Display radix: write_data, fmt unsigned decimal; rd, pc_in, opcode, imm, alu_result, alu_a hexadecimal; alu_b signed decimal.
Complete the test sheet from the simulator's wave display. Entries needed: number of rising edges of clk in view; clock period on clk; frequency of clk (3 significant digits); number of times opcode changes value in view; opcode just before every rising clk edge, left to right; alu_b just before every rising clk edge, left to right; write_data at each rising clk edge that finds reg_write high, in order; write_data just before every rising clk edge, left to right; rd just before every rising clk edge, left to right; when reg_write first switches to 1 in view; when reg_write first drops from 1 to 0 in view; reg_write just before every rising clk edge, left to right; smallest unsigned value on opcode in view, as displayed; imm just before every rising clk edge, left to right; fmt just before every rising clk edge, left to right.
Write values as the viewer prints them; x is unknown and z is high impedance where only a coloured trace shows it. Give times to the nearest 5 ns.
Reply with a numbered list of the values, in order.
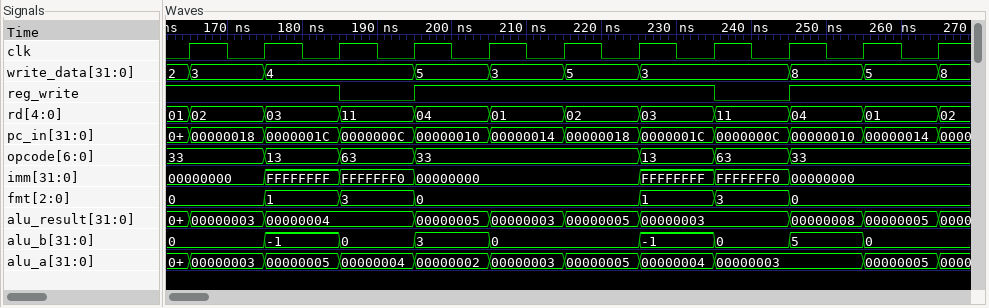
1. 11
2. 10 ns
3. 100 MHz
4. 6
5. 33, 33, 13, 63, 33, 33, 33, 13, 63, 33, 33
6. 0, 0, -1, 0, 3, 0, 0, -1, 0, 5, 0
7. 2, 3, 4, 5, 3, 5, 3, 8, 5
8. 2, 3, 4, 4, 5, 3, 5, 3, 3, 8, 5
9. 01, 02, 03, 11, 04, 01, 02, 03, 11, 04, 01
10. 195 ns
11. 185 ns
12. 1 1 1 0 1 1 1 1 0 1 1
13. 13
14. 00000000, 00000000, FFFFFFFF, FFFFFFF0, 00000000, 00000000, 00000000, FFFFFFFF, FFFFFFF0, 00000000, 00000000
15. 0, 0, 1, 3, 0, 0, 0, 1, 3, 0, 0
